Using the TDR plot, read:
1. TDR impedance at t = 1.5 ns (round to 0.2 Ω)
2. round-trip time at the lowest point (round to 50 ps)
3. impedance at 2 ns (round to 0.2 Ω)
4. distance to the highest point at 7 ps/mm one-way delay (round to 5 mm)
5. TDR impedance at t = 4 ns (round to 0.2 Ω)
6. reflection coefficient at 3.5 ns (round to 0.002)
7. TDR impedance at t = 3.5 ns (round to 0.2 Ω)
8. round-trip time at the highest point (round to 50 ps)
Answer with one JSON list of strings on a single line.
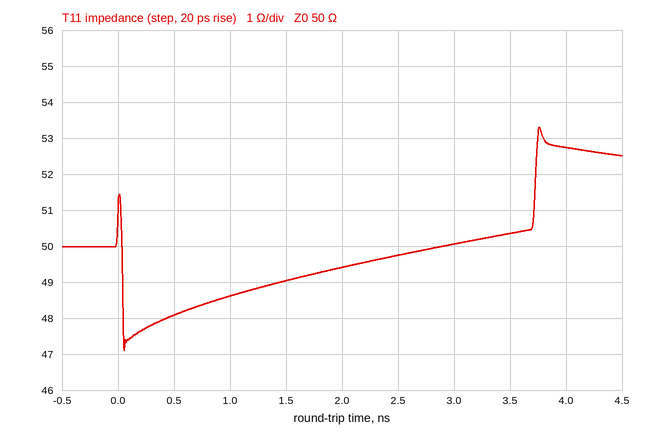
["49.0 Ω", "50 ps", "49.4 Ω", "270 mm", "52.8 Ω", "+0.004", "50.4 Ω", "3.75 ns"]
